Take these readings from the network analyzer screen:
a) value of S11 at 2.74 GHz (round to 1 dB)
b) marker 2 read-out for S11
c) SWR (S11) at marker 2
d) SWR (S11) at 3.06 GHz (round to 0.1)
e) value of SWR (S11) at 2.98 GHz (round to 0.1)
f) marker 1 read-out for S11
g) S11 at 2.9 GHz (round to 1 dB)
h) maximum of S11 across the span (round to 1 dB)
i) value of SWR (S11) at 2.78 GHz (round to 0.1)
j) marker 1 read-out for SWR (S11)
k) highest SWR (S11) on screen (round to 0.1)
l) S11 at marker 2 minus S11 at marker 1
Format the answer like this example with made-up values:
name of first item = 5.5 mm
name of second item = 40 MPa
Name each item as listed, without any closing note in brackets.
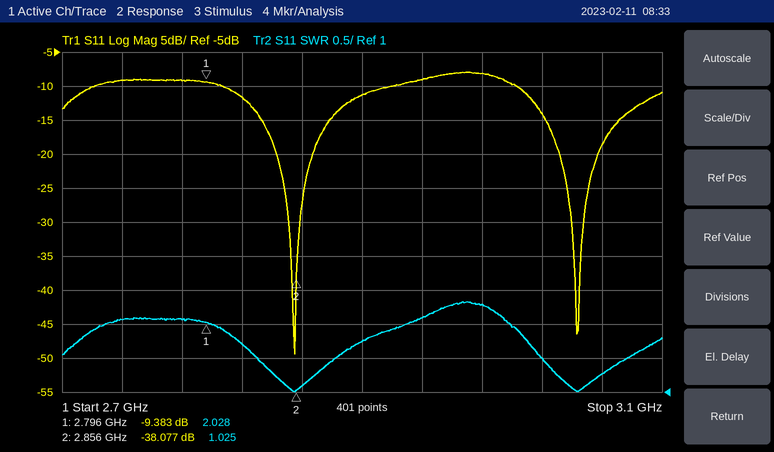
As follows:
value of S11 at 2.74 GHz = -9 dB
marker 2 read-out for S11 = -38.077 dB
SWR (S11) at marker 2 = 1.025
SWR (S11) at 3.06 GHz = 1.3
value of SWR (S11) at 2.98 GHz = 2.3
marker 1 read-out for S11 = -9.383 dB
S11 at 2.9 GHz = -11 dB
maximum of S11 across the span = -8 dB
value of SWR (S11) at 2.78 GHz = 2.1
marker 1 read-out for SWR = 2.028
highest SWR (S11) on screen = 2.3
S11 at marker 2 minus S11 at marker 1 = -28.694 dB
